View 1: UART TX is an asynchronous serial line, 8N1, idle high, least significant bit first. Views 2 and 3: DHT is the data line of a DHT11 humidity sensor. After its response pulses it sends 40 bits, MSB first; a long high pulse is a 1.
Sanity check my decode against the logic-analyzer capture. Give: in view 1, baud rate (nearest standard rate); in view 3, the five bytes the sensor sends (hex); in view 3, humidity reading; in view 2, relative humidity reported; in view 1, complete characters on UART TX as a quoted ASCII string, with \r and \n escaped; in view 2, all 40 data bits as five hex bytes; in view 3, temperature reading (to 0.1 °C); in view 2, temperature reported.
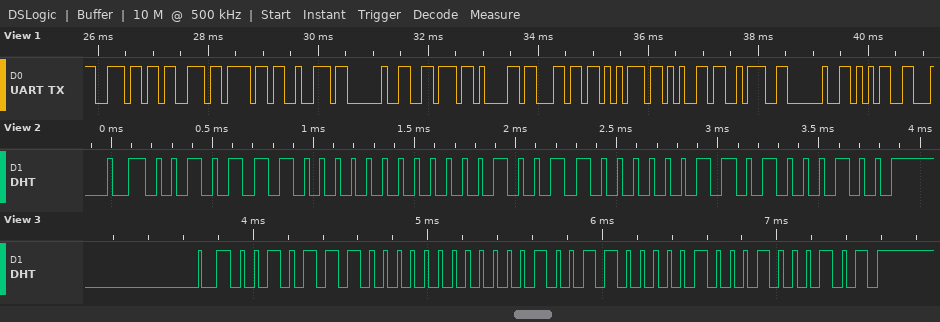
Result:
9600 baud
2E 00 13 04 45
46 %
46 %
"nsor value: 5"
2E 00 13 03 44
19.4 °C
19.3 °C
